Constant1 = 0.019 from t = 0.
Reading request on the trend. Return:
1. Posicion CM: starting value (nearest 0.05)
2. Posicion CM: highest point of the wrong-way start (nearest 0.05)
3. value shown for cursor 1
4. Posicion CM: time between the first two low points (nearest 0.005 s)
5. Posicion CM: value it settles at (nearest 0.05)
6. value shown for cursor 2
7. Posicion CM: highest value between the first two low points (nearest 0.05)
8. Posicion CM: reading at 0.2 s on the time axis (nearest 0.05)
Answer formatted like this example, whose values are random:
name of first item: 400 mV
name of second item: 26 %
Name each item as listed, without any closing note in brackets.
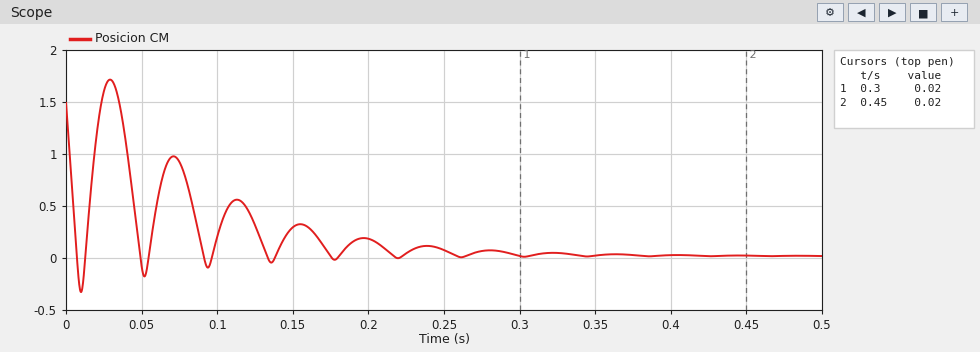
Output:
Posicion CM: starting value: 1.50
Posicion CM: highest point of the wrong-way start: 1.70
value shown for cursor 1: 0.02
Posicion CM: time between the first two low points: 0.040 s
Posicion CM: value it settles at: 0.00
value shown for cursor 2: 0.02
Posicion CM: highest value between the first two low points: 1.70
Posicion CM: reading at 0.2 s on the time axis: 0.20
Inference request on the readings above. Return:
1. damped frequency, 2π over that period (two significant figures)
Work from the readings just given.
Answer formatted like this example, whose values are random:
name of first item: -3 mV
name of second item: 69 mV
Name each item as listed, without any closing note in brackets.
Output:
damped frequency, 2π over that period: 160 rad/s
